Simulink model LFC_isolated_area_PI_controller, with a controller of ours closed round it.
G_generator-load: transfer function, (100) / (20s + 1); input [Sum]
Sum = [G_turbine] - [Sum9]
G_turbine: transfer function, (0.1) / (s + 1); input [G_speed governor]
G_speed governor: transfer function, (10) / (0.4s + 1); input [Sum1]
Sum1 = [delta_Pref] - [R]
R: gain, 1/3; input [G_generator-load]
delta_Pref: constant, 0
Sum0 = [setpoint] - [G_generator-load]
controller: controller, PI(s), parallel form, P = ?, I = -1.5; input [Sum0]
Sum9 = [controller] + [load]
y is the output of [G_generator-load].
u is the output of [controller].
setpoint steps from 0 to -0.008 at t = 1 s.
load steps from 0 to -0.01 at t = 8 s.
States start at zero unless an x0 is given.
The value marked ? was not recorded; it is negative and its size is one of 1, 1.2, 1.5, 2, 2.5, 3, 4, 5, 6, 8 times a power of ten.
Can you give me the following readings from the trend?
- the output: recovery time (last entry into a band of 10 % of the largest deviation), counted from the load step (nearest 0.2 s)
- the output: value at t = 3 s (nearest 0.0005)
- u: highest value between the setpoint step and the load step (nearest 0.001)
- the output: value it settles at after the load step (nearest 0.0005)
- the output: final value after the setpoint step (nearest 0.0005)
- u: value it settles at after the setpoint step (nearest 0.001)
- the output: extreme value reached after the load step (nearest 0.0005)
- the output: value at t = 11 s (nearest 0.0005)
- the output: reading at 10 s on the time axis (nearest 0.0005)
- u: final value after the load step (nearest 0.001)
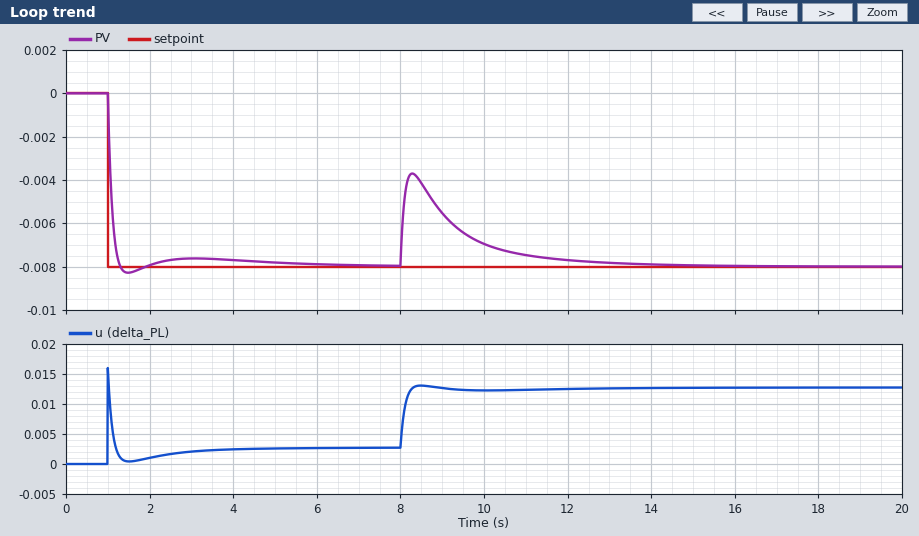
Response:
3.4 s
-0.0075
0.016
-0.0080
-0.0080
0.003
-0.0035
-0.0075
-0.0070
0.013
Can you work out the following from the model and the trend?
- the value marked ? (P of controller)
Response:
-2
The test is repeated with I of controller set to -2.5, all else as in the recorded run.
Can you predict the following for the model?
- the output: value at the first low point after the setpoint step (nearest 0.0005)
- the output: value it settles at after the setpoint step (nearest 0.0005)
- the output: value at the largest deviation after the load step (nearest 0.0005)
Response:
-0.0085
-0.0080
-0.0040
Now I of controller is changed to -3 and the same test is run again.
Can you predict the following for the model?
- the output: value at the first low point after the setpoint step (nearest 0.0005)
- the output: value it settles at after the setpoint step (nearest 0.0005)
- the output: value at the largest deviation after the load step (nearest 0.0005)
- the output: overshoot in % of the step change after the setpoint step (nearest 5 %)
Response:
-0.0085
-0.0080
-0.0040
10 %
